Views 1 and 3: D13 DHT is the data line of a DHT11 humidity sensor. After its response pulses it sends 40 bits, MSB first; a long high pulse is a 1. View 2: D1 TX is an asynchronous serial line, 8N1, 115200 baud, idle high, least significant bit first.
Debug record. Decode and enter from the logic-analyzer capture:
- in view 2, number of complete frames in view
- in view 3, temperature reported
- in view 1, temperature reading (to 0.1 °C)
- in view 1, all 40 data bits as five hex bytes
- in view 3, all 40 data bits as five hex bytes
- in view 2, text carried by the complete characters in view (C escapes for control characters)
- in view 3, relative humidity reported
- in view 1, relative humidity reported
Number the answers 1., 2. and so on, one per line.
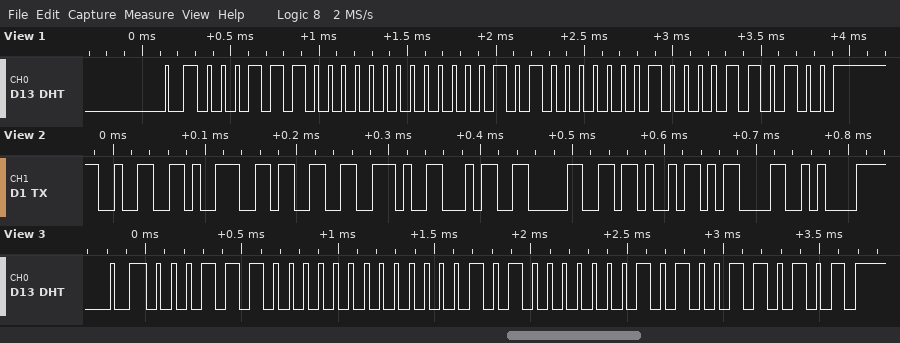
1. 9
2. 20.5 °C
3. 20.4 °C
4. 1C 00 14 04 34
5. 1C 00 14 05 35
6. "293.40K\r\n"
7. 28 %
8. 28 %
